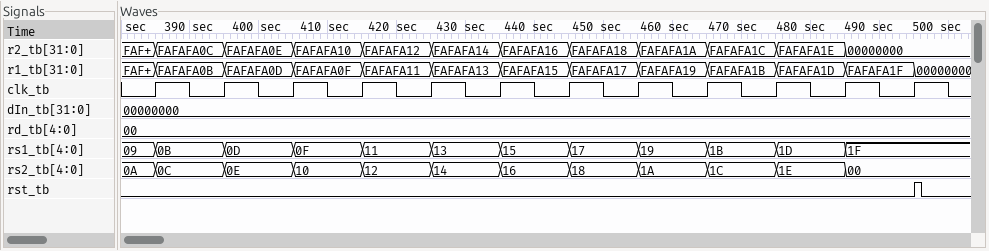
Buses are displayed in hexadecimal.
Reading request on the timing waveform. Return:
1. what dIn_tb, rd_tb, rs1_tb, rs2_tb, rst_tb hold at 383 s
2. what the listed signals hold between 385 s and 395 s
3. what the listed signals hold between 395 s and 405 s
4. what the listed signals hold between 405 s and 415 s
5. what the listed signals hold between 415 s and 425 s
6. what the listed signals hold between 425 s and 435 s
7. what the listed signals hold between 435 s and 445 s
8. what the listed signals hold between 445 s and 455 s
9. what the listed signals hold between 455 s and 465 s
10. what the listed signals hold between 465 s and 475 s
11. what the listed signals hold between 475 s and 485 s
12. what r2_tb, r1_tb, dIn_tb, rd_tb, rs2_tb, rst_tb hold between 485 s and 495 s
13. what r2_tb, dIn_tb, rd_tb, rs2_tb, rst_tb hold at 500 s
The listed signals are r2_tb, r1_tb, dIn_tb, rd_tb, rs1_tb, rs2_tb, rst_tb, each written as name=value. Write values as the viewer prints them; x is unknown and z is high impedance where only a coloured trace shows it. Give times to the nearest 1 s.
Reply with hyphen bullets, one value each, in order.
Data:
- dIn_tb=00000000, rd_tb=00, rs1_tb=09, rs2_tb=0A, rst_tb=0
- r2_tb=FAFAFA0C, r1_tb=FAFAFA0B, dIn_tb=00000000, rd_tb=00, rs1_tb=0B, rs2_tb=0C, rst_tb=0
- r2_tb=FAFAFA0E, r1_tb=FAFAFA0D, dIn_tb=00000000, rd_tb=00, rs1_tb=0D, rs2_tb=0E, rst_tb=0
- r2_tb=FAFAFA10, r1_tb=FAFAFA0F, dIn_tb=00000000, rd_tb=00, rs1_tb=0F, rs2_tb=10, rst_tb=0
- r2_tb=FAFAFA12, r1_tb=FAFAFA11, dIn_tb=00000000, rd_tb=00, rs1_tb=11, rs2_tb=12, rst_tb=0
- r2_tb=FAFAFA14, r1_tb=FAFAFA13, dIn_tb=00000000, rd_tb=00, rs1_tb=13, rs2_tb=14, rst_tb=0
- r2_tb=FAFAFA16, r1_tb=FAFAFA15, dIn_tb=00000000, rd_tb=00, rs1_tb=15, rs2_tb=16, rst_tb=0
- r2_tb=FAFAFA18, r1_tb=FAFAFA17, dIn_tb=00000000, rd_tb=00, rs1_tb=17, rs2_tb=18, rst_tb=0
- r2_tb=FAFAFA1A, r1_tb=FAFAFA19, dIn_tb=00000000, rd_tb=00, rs1_tb=19, rs2_tb=1A, rst_tb=0
- r2_tb=FAFAFA1C, r1_tb=FAFAFA1B, dIn_tb=00000000, rd_tb=00, rs1_tb=1B, rs2_tb=1C, rst_tb=0
- r2_tb=FAFAFA1E, r1_tb=FAFAFA1D, dIn_tb=00000000, rd_tb=00, rs1_tb=1D, rs2_tb=1E, rst_tb=0
- r2_tb=00000000, r1_tb=FAFAFA1F, dIn_tb=00000000, rd_tb=00, rs2_tb=00, rst_tb=0
- r2_tb=00000000, dIn_tb=00000000, rd_tb=00, rs2_tb=00, rst_tb=0
